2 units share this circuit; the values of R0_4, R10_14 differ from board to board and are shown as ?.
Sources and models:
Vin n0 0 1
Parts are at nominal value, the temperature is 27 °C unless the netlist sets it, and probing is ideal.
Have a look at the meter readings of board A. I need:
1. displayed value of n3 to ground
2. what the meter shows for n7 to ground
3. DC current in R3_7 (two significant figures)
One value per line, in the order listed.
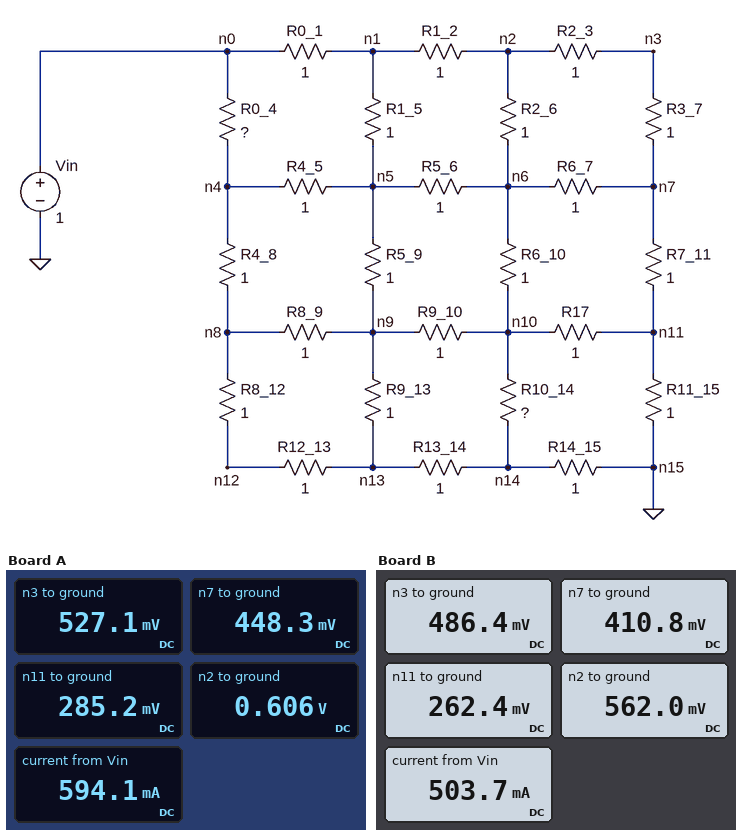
527.1 mV
448.3 mV
79 mA
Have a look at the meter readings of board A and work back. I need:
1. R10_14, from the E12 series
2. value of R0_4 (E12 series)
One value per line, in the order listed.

0.68 Ω
0.47 Ω
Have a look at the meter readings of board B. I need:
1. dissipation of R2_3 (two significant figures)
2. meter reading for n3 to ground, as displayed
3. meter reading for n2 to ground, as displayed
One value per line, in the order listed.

5.7 mW
486.4 mV
562.0 mV
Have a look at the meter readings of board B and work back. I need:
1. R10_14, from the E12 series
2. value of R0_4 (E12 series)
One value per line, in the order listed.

1.5 Ω
1.5 Ω
